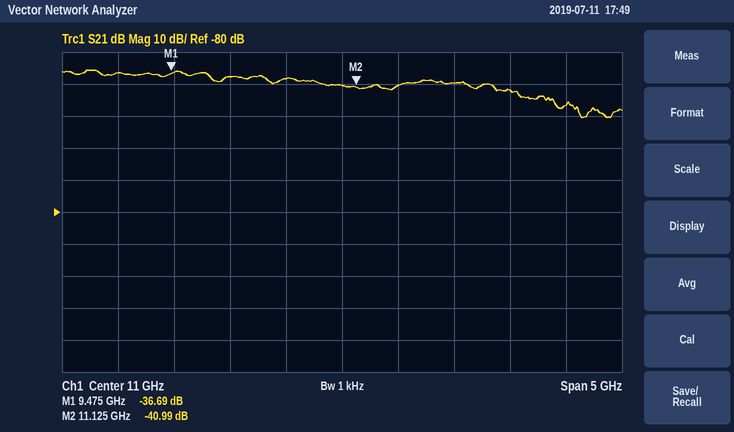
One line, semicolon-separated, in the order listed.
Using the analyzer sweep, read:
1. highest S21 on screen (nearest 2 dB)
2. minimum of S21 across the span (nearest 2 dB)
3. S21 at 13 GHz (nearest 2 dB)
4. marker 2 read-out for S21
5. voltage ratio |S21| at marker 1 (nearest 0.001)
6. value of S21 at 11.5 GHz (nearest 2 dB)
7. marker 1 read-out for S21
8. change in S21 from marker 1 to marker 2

-36 dB; -50 dB; -46 dB; -40.99 dB; 0.015; -40 dB; -36.69 dB; -4.30 dB
